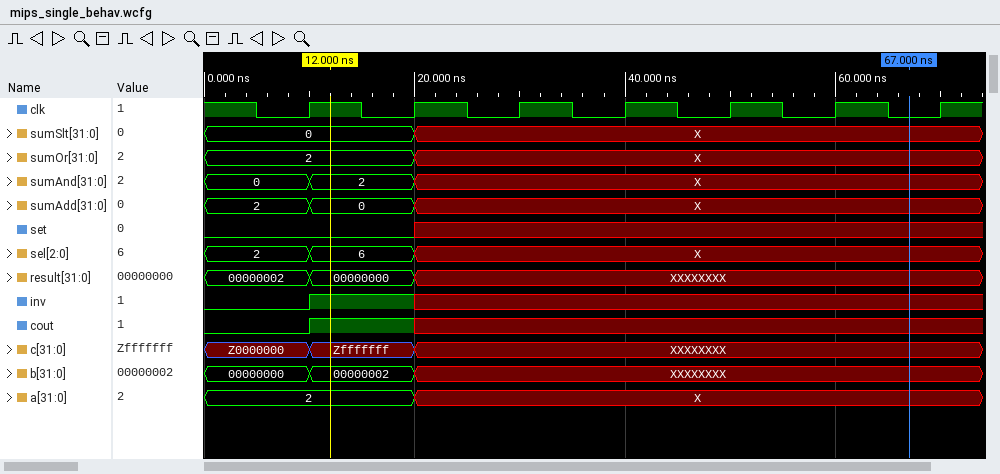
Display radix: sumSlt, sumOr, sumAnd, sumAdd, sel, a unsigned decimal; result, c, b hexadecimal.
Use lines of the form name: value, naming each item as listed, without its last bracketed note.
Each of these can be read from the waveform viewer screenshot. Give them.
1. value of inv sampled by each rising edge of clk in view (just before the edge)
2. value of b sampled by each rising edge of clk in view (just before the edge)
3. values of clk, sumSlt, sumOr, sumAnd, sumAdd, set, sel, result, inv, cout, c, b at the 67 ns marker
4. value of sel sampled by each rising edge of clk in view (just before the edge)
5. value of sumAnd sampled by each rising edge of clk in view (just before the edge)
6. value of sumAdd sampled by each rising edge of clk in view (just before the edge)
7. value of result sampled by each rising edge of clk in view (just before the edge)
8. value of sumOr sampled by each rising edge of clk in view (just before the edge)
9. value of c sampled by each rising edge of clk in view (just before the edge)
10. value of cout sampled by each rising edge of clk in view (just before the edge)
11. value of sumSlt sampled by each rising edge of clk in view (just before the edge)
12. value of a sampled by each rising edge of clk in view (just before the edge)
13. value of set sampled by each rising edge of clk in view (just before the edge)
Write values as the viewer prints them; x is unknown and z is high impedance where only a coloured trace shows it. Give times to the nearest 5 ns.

value of inv sampled by each rising edge of clk in view: 0 1 x x x x x
value of b sampled by each rising edge of clk in view: 00000000, 00000002, XXXXXXXX, XXXXXXXX, XXXXXXXX, XXXXXXXX, XXXXXXXX
values of clk, sumSlt, sumOr, sumAnd, sumAdd, set, sel, result, inv, cout, c, b at the 67 ns marker: clk=0, sumSlt=X, sumOr=X, sumAnd=X, sumAdd=X, set=x, sel=X, result=XXXXXXXX, inv=x, cout=x, c=XXXXXXXX, b=XXXXXXXX
value of sel sampled by each rising edge of clk in view: 2, 6, X, X, X, X, X
value of sumAnd sampled by each rising edge of clk in view: 0, 2, X, X, X, X, X
value of sumAdd sampled by each rising edge of clk in view: 2, 0, X, X, X, X, X
value of result sampled by each rising edge of clk in view: 00000002, 00000000, XXXXXXXX, XXXXXXXX, XXXXXXXX, XXXXXXXX, XXXXXXXX
value of sumOr sampled by each rising edge of clk in view: 2, 2, X, X, X, X, X
value of c sampled by each rising edge of clk in view: Z0000000, Zfffffff, XXXXXXXX, XXXXXXXX, XXXXXXXX, XXXXXXXX, XXXXXXXX
value of cout sampled by each rising edge of clk in view: 0 1 x x x x x
value of sumSlt sampled by each rising edge of clk in view: 0, 0, X, X, X, X, X
value of a sampled by each rising edge of clk in view: 2, 2, X, X, X, X, X
value of set sampled by each rising edge of clk in view: 0 0 x x x x x
